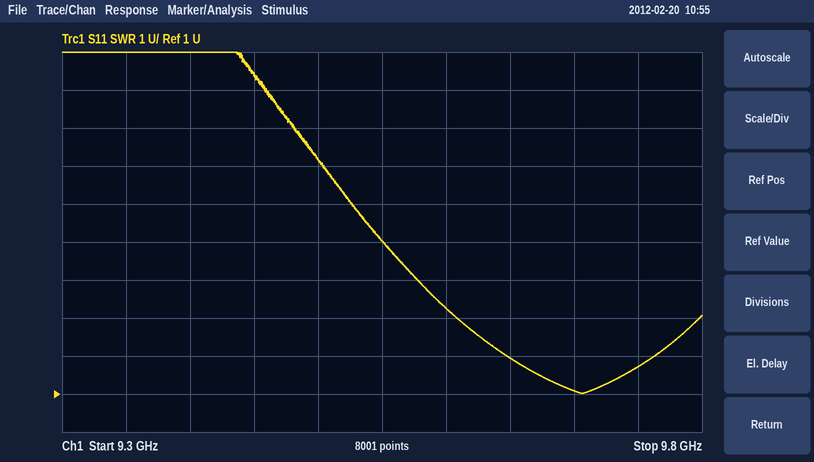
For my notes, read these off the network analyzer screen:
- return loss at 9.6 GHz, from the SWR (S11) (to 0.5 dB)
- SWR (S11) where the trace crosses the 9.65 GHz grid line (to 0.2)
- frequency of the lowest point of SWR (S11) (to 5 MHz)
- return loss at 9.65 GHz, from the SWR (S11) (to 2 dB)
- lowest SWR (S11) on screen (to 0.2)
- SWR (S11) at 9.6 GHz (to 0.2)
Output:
5.5 dB
2.0
9.705 GHz
10 dB
1.0
3.2
